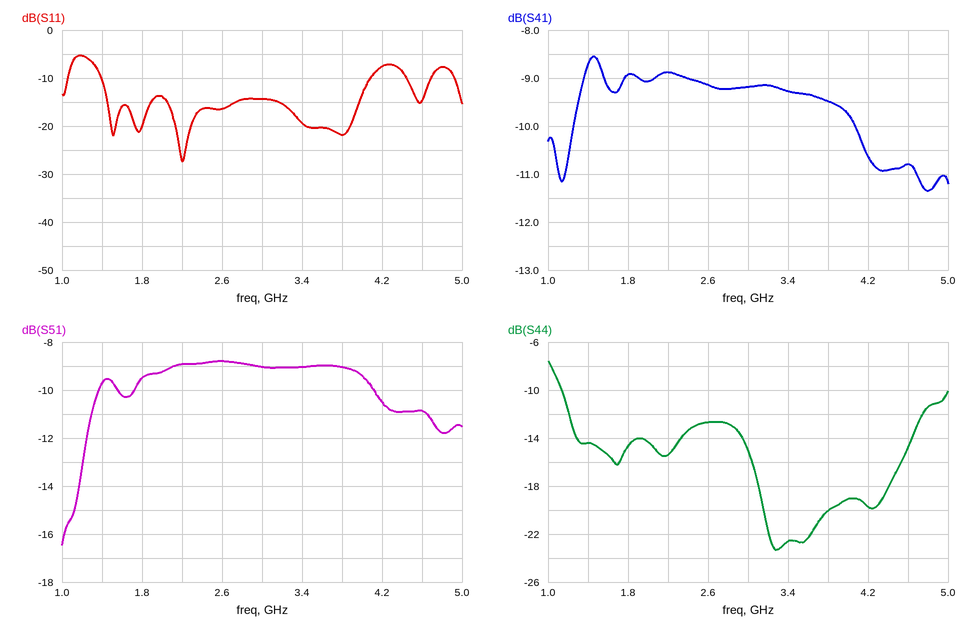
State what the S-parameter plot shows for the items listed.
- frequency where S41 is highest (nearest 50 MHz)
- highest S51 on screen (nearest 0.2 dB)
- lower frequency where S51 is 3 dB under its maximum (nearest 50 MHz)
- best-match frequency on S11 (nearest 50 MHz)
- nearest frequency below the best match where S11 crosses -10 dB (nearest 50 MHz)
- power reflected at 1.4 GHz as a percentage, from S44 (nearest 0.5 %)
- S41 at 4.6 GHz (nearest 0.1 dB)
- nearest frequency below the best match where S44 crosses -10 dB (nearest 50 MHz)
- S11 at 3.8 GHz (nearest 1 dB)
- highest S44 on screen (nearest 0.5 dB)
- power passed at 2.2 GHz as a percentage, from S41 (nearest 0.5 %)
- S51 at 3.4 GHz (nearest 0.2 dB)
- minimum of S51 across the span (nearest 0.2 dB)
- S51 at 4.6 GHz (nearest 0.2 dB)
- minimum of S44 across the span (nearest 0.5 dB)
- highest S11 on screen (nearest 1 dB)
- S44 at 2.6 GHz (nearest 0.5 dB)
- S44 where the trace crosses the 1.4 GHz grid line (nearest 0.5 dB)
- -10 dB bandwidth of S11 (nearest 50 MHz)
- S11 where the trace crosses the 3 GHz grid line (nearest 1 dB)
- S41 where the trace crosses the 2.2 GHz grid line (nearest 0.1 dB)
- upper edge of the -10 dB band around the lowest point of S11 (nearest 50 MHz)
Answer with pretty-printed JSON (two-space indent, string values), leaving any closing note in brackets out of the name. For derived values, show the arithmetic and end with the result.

{
  "frequency where S41 is highest": "1.45 GHz",
  "highest S51 on screen": "-8.8 dB",
  "lower frequency where S51 is 3 dB under its maximum": "1.25 GHz",
  "best-match frequency on S11": "2.20 GHz",
  "nearest frequency below the best match where S11 crosses -10 dB": "1.40 GHz",
  "power reflected at 1.4 GHz as a percentage, from S44": "10^(-14.5/10) ≈ 3.5 %",
  "S41 at 4.6 GHz": "-10.8 dB",
  "nearest frequency below the best match where S44 crosses -10 dB": "1.15 GHz",
  "S11 at 3.8 GHz": "-22 dB",
  "highest S44 on screen": "-7.5 dB",
  "power passed at 2.2 GHz as a percentage, from S41": "10^(-8.9/10) ≈ 12.9 %, so 13.0 % to the nearest 0.5 %",
  "S51 at 3.4 GHz": "-9.0 dB",
  "minimum of S51 across the span": "-16.4 dB",
  "S51 at 4.6 GHz": "-10.8 dB",
  "minimum of S44 across the span": "-23.5 dB",
  "highest S11 on screen": "-5 dB",
  "S44 at 2.6 GHz": "-12.5 dB",
  "S44 where the trace crosses the 1.4 GHz grid line": "-14.5 dB",
  "-10 dB bandwidth of S11": "4.10 GHz − 1.40 GHz = 2.70 GHz",
  "S11 where the trace crosses the 3 GHz grid line": "-14 dB",
  "S41 where the trace crosses the 2.2 GHz grid line": "-8.9 dB",
  "upper edge of the -10 dB band around the lowest point of S11": "4.10 GHz"
}
